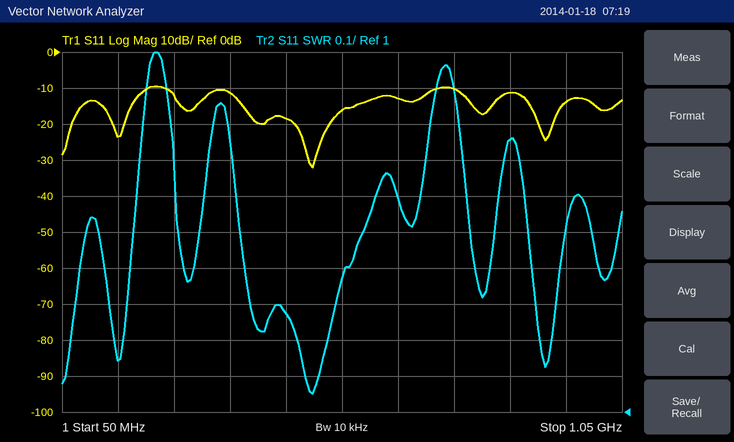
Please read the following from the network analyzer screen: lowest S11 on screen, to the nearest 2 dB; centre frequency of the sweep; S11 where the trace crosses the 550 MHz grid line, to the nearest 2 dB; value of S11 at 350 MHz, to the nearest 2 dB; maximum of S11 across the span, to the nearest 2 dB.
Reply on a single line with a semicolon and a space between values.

-32 dB; 550 MHz; -16 dB; -12 dB; -10 dB
